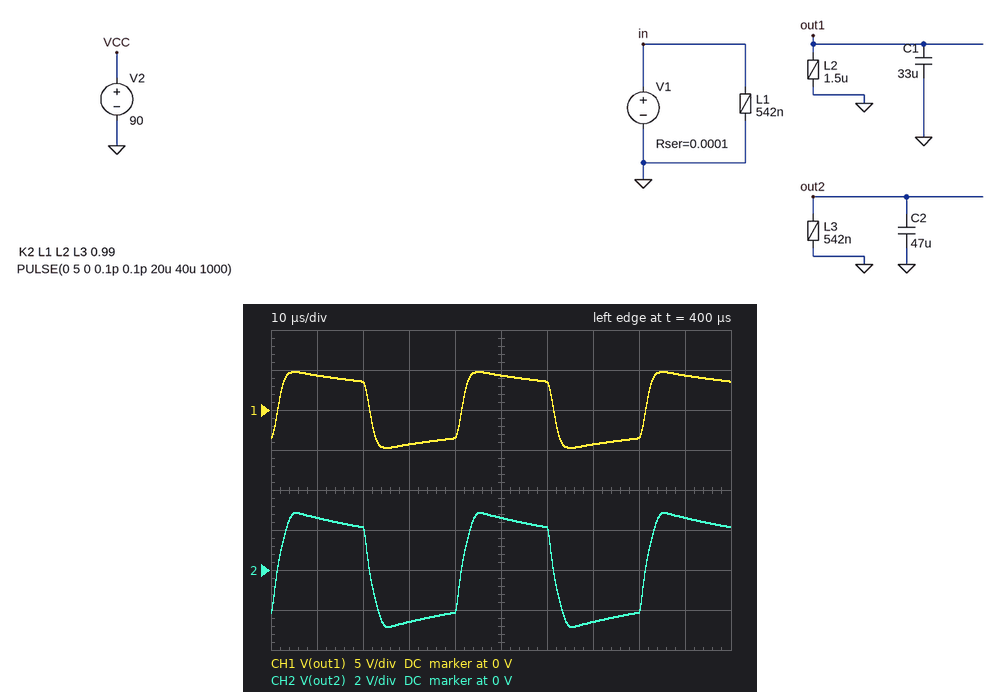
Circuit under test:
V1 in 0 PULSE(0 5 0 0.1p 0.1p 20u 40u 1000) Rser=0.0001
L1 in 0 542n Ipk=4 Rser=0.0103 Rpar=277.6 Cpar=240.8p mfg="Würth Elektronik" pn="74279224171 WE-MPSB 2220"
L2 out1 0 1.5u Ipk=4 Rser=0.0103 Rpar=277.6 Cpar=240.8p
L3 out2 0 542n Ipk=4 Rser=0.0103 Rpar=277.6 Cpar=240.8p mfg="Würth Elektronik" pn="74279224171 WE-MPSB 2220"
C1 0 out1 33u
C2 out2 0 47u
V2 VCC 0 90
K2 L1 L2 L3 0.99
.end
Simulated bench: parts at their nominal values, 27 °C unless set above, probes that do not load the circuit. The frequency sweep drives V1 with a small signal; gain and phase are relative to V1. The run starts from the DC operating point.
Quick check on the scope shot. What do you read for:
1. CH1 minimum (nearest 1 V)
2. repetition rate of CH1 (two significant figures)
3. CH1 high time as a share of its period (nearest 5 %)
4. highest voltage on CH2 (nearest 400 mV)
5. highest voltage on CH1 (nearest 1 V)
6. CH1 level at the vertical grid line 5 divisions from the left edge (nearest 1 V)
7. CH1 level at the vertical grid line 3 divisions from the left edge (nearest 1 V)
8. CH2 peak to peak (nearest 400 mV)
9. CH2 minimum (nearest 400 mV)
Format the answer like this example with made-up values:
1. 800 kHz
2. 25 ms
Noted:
1. -5 V
2. 25 kHz
3. 50 %
4. 2.8 V
5. 5 V
6. 4 V
7. -4 V
8. 5.6 V
9. -2.8 V
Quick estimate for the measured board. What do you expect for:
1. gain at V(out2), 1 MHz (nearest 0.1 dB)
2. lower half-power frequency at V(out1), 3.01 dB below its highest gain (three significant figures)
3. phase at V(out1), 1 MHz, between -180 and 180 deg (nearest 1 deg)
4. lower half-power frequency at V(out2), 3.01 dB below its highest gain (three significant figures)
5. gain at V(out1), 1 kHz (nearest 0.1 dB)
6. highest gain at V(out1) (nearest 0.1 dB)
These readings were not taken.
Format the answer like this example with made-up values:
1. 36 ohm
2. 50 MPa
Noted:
1. -29.7 dB
2. 3.03 kHz
3. -170 deg
4. 3.00 kHz
5. -5.8 dB
6. 4.4 dB
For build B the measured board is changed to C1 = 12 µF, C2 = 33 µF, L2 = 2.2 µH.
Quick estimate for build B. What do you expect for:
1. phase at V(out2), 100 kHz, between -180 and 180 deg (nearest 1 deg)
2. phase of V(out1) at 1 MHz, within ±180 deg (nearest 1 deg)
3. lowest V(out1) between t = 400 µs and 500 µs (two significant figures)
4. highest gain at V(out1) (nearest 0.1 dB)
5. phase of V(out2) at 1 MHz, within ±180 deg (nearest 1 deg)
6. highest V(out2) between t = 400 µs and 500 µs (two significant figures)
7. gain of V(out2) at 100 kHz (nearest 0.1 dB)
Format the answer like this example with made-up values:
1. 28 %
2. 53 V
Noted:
1. -45 deg
2. -172 deg
3. -6.8 V
4. 6.4 dB
5. -157 deg
6. 3.3 V
7. -0.2 dB
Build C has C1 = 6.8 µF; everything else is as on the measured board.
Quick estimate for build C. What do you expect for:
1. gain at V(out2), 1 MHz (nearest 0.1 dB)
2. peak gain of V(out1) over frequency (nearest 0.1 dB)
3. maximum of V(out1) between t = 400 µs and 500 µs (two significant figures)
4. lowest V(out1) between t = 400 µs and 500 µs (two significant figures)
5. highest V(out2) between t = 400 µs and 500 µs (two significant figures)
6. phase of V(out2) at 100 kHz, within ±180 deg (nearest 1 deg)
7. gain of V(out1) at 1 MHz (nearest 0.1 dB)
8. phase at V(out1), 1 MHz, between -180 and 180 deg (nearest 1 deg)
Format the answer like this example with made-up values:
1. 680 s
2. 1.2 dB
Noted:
1. -30.4 dB
2. 4.4 dB
3. 5.3 V
4. -5.3 V
5. 3.1 V
6. -43 deg
7. -16.1 dB
8. -169 deg
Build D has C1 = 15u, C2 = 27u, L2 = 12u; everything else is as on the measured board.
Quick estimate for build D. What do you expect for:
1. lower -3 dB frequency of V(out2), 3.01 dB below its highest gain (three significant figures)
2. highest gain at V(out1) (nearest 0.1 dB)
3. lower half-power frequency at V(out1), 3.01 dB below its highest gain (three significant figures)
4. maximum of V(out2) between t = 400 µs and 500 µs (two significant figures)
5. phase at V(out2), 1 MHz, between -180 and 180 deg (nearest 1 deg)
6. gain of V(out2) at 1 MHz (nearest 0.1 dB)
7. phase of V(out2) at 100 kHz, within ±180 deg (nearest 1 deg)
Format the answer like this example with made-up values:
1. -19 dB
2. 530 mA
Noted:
1. 2.90 kHz
2. 13.5 dB
3. 2.95 kHz
4. 2.6 V
5. -156 deg
6. -24.3 dB
7. -93 deg
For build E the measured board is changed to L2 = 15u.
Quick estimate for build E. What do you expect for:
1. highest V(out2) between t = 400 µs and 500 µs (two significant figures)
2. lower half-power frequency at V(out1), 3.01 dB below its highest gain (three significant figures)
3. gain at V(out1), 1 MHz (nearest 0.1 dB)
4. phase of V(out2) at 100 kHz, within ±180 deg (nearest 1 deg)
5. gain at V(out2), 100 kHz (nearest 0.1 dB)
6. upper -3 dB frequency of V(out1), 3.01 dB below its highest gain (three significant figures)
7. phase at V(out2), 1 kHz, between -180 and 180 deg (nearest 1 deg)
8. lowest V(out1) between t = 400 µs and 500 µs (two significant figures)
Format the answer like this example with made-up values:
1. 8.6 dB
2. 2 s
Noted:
1. 1.9 V
2. 2.67 kHz
3. -41.3 dB
4. 32 deg
5. -16.1 dB
6. 19.5 kHz
7. 71 deg
8. -10 V
